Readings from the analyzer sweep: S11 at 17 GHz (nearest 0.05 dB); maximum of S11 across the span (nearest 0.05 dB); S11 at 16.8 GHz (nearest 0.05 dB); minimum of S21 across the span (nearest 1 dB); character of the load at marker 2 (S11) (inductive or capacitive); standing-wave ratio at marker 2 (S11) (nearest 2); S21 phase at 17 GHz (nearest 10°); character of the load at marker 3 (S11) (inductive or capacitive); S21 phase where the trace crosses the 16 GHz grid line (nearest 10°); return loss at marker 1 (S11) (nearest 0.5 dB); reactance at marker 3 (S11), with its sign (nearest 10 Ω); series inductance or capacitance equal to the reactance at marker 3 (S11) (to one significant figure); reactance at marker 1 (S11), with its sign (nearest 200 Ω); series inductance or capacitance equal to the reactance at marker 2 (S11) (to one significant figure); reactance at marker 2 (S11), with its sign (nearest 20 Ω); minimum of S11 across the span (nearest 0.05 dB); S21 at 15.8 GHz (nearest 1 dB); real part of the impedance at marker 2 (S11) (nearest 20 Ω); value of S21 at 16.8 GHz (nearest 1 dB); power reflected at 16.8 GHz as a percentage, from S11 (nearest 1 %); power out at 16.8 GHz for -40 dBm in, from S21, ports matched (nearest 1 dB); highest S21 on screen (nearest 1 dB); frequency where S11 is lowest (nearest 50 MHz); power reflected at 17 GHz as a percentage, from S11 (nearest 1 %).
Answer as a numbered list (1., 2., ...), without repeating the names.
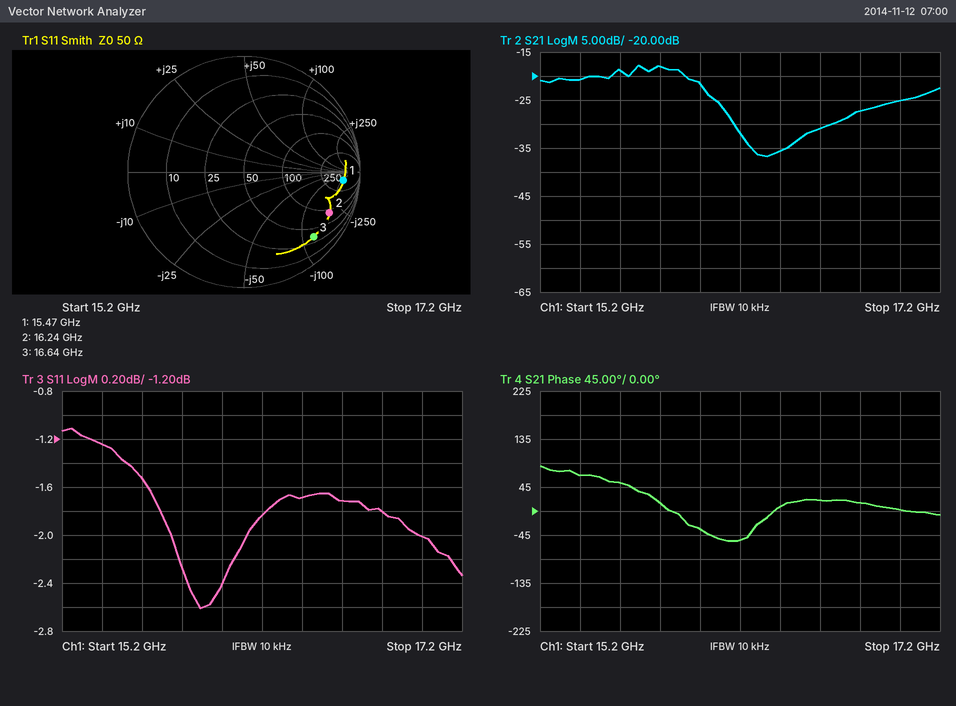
1. -2.00 dB
2. -1.10 dB
3. -1.80 dB
4. -37 dB
5. capacitive
6. 10
7. 0°
8. capacitive
9. -30°
10. 1.5 dB
11. -120 Ω
12. 80 fF
13. -200 Ω
14. 50 fF
15. -180 Ω
16. -2.60 dB
17. -18 dB
18. 80 Ω
19. -27 dB
20. 66 %
21. -67 dBm
22. -18 dB
23. 15.90 GHz
24. 63 %
